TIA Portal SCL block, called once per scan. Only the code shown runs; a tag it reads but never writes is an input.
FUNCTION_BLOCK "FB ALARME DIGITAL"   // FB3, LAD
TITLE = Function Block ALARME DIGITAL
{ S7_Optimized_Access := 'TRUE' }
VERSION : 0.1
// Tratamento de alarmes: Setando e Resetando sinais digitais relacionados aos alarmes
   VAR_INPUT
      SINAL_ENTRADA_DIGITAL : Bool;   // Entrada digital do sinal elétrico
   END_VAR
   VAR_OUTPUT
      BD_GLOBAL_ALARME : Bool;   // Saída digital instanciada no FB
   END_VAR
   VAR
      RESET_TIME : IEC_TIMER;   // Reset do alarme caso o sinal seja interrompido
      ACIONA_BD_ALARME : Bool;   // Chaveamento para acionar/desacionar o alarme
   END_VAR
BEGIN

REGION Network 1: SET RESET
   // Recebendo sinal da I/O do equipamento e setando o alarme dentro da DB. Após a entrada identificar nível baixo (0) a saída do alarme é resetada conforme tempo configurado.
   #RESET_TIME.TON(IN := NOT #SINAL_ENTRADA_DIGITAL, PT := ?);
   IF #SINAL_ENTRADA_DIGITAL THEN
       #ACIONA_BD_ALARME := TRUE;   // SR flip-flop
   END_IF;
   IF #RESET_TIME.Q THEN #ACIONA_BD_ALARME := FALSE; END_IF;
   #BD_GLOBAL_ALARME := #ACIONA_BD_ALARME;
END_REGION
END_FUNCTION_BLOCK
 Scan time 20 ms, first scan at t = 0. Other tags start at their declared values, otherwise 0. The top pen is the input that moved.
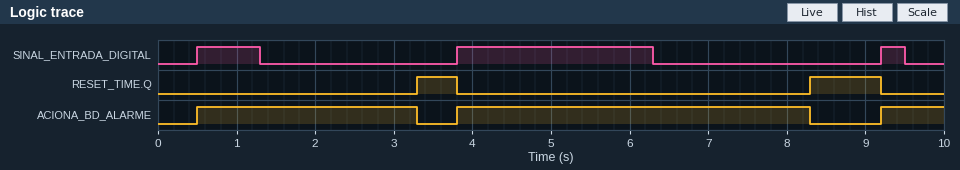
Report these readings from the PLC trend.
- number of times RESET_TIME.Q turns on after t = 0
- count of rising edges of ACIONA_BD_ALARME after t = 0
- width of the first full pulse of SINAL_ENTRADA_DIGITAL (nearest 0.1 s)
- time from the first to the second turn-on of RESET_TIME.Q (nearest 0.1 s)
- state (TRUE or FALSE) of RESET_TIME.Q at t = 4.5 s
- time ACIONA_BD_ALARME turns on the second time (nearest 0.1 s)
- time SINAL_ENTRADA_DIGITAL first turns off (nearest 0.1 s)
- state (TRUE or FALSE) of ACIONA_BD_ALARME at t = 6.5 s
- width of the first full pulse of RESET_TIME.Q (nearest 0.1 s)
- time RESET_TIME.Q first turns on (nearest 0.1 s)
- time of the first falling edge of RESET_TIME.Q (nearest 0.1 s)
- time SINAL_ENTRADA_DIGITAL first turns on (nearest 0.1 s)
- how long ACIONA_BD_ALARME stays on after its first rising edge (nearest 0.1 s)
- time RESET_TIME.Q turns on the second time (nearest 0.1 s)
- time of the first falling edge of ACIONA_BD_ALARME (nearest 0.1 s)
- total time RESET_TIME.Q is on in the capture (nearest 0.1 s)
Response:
2
3
0.8 s
5.0 s
FALSE
3.8 s
1.3 s
TRUE
0.5 s
3.3 s
3.8 s
0.5 s
2.8 s
8.3 s
3.3 s
1.4 s
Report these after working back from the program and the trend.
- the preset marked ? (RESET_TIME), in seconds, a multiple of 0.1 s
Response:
2.0 s
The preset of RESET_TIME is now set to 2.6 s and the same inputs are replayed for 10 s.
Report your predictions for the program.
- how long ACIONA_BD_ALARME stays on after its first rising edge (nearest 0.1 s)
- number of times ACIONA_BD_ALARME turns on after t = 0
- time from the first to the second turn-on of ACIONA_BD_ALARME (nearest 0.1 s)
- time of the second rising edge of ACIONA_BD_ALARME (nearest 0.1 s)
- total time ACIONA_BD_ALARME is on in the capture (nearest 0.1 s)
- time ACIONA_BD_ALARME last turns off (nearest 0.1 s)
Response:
8.4 s
2
8.7 s
9.2 s
9.2 s
8.9 s
